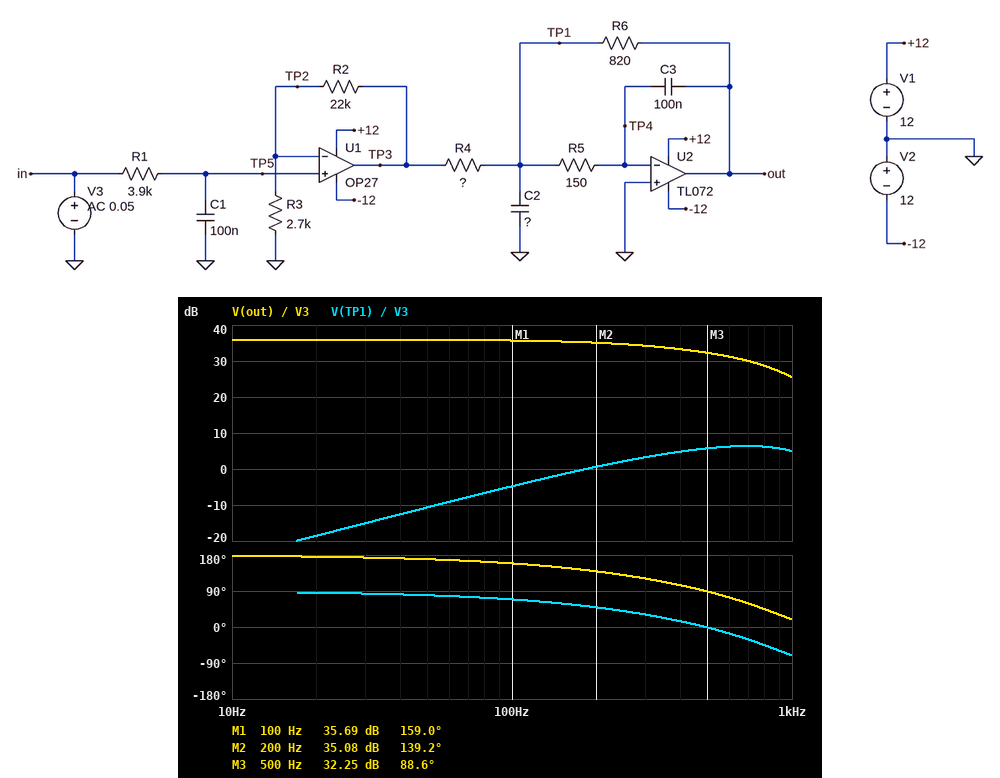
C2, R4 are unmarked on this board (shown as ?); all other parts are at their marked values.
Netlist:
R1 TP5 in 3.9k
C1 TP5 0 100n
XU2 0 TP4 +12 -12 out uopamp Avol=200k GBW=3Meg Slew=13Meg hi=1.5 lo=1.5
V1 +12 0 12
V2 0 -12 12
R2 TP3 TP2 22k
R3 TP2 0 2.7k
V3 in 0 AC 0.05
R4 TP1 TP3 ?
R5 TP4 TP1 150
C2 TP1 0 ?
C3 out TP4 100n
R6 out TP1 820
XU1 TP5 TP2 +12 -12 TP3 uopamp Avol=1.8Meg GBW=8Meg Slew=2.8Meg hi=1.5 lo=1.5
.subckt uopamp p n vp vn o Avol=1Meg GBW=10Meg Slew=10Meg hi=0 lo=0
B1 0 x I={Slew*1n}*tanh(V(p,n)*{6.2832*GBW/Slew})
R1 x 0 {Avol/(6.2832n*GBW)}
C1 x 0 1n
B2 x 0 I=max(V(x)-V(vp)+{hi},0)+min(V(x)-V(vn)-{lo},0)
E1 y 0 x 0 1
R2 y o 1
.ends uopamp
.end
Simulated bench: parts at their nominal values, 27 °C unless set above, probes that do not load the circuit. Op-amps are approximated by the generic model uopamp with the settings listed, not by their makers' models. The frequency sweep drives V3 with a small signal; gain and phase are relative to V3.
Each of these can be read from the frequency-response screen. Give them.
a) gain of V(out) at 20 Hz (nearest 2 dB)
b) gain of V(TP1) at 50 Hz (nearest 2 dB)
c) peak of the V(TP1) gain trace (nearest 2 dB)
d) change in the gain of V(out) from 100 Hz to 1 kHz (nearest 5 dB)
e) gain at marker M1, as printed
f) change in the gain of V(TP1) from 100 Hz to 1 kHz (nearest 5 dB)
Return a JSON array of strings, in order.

["36 dB", "-10 dB", "6 dB", "-10 dB", "35.69 dB", "10 dB"]
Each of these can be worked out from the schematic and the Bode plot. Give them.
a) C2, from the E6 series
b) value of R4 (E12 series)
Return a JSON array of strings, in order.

["2.2 µF", "120 Ω"]
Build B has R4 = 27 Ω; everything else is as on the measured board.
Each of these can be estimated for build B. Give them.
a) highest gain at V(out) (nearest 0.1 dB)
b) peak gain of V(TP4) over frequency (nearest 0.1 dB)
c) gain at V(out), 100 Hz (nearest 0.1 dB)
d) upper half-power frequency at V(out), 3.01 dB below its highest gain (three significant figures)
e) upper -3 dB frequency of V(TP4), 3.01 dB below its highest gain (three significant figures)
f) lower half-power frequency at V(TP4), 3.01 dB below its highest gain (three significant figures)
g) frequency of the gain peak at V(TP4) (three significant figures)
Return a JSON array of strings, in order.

["48.9 dB", "-35.7 dB", "48.2 dB", "228 Hz", "835 Hz", "146 Hz", "355 Hz"]
